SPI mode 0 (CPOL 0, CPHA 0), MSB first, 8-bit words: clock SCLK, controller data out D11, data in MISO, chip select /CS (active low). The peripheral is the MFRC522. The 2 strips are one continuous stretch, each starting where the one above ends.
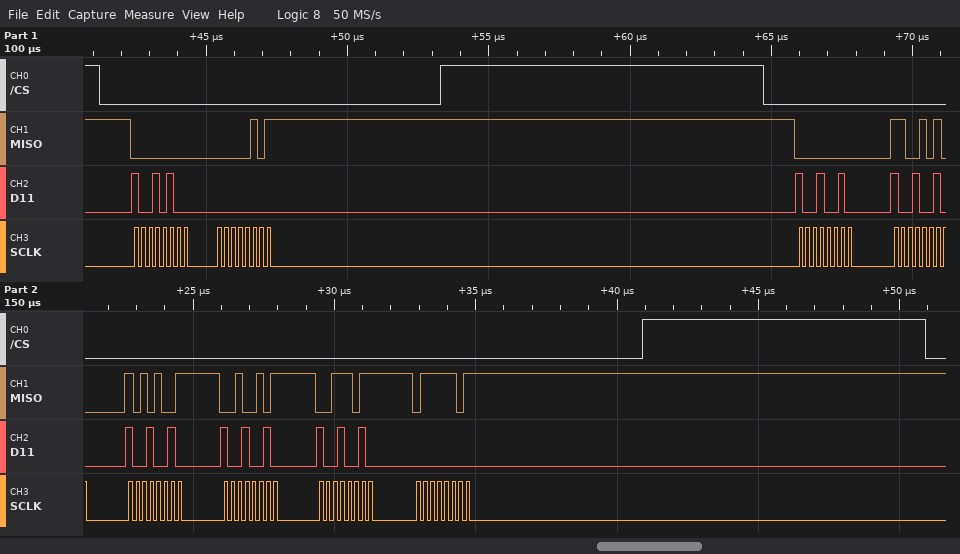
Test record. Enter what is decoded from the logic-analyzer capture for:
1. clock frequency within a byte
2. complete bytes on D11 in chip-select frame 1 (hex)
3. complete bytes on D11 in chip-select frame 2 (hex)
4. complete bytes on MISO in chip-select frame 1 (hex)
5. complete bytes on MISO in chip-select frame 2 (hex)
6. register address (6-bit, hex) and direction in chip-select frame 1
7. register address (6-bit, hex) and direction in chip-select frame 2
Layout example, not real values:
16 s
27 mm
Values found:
4 MHz
0x94 0x00
0x92 0x92 0x92 0x92 0x92 0x00
0x00 0x05
0x00 0xCA 0xA9 0x25 0x3B 0x7D
0x0A read
0x09 read
